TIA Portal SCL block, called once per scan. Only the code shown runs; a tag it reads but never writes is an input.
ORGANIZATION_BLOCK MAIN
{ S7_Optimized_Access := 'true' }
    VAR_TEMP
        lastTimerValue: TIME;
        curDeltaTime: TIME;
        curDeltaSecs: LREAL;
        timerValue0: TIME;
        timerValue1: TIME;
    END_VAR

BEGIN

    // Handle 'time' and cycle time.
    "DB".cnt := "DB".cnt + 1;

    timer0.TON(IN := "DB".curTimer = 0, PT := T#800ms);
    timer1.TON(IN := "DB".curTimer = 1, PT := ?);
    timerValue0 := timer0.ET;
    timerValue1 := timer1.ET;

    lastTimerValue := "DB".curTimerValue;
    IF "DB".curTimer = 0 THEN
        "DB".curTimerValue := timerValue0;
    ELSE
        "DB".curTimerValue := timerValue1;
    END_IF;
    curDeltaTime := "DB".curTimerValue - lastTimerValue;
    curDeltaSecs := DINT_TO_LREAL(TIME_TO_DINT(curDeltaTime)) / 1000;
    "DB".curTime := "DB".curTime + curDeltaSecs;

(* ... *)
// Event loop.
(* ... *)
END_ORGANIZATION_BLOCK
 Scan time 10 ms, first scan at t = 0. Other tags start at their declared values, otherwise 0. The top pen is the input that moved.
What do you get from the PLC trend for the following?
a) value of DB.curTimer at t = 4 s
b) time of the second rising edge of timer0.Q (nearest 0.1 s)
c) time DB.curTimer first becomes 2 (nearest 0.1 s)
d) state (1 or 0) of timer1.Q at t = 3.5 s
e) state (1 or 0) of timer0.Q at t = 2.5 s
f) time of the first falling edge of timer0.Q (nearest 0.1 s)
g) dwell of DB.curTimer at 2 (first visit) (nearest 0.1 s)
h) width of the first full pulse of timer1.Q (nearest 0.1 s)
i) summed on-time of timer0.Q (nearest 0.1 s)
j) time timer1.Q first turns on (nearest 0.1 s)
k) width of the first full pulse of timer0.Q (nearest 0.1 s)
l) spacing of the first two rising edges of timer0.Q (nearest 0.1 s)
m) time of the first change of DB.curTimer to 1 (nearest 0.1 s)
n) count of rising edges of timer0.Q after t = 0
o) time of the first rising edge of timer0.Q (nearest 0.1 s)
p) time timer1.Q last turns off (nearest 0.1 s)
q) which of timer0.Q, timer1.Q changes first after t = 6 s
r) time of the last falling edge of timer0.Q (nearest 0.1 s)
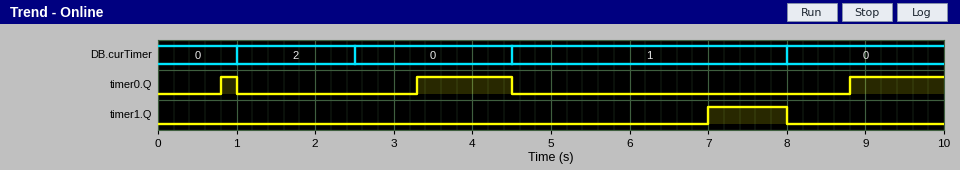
0
3.3 s
1.0 s
0
0
1.0 s
1.5 s
1.0 s
2.6 s
7.0 s
0.2 s
2.5 s
4.5 s
3
0.8 s
8.0 s
timer1.Q
4.5 s
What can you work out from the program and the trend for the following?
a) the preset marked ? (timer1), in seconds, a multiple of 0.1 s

2.5 s
